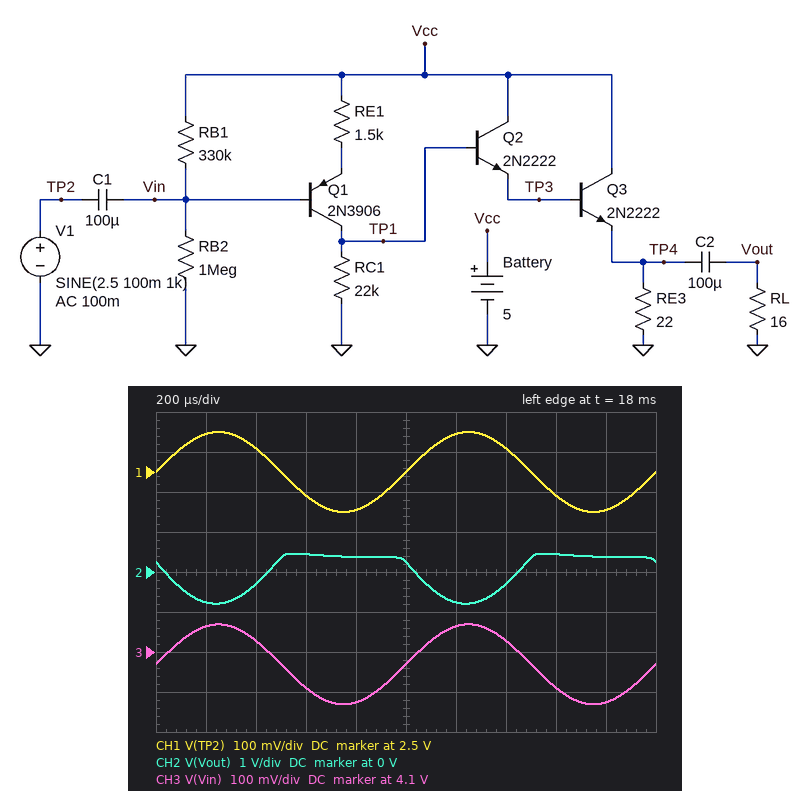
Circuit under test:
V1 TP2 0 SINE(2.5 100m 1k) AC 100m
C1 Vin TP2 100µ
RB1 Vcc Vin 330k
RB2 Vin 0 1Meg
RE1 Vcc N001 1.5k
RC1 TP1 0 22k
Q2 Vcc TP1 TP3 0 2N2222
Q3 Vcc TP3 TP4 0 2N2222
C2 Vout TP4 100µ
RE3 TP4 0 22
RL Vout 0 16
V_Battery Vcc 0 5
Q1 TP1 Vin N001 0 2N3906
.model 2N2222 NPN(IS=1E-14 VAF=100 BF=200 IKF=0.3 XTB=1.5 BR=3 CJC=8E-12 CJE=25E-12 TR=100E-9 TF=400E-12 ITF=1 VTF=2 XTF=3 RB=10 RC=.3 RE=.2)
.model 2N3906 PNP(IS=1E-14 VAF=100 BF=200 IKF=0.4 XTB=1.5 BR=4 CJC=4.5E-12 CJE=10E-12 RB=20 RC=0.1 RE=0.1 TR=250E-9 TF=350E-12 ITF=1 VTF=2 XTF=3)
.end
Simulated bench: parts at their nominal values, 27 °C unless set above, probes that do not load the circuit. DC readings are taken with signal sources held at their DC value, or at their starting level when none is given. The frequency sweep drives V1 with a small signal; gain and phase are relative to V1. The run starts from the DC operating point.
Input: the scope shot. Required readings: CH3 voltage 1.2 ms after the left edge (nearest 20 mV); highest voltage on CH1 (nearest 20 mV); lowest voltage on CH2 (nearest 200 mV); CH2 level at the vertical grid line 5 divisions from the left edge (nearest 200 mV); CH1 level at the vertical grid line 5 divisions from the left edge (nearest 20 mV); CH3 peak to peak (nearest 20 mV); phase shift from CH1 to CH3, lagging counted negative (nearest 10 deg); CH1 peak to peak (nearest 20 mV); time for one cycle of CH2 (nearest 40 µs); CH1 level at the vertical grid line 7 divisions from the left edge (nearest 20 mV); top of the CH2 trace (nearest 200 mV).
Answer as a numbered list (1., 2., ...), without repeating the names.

1. 4.16 V
2. 2.60 V
3. -800 mV
4. 200 mV
5. 2.50 V
6. 200 mV
7. 0 deg
8. 200 mV
9. 1.00 ms
10. 2.56 V
11. 400 mV
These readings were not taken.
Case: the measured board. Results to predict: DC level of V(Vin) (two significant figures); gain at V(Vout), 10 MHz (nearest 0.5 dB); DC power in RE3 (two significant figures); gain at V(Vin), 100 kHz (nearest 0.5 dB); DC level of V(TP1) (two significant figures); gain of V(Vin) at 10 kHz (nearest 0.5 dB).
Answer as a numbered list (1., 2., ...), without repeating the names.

1. 4.1 V
2. -3.5 dB
3. 420 mW
4. 0 dB
5. 4.5 V
6. 0 dB
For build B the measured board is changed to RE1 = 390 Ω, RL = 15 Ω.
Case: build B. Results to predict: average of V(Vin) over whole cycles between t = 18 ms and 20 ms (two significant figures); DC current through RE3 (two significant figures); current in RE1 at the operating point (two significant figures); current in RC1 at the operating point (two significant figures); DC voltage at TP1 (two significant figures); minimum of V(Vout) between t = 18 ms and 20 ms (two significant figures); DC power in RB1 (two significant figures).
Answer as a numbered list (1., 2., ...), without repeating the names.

1. 4.3 V
2. 150 mA
3. 230 µA
4. 220 µA
5. 4.8 V
6. -1.1 V
7. 1.5 µW
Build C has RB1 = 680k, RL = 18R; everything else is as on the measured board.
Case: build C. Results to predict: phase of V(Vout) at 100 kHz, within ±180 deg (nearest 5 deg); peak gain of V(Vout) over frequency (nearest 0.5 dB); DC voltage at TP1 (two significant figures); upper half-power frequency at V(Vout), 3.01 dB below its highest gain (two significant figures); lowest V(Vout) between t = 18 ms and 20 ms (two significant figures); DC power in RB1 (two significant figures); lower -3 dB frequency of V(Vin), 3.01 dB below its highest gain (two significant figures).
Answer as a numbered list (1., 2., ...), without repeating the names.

1. 155 deg
2. 11.5 dB
3. 4.6 V
4. 280 kHz
5. -770 mV
6. 1.3 µW
7. 520 mHz
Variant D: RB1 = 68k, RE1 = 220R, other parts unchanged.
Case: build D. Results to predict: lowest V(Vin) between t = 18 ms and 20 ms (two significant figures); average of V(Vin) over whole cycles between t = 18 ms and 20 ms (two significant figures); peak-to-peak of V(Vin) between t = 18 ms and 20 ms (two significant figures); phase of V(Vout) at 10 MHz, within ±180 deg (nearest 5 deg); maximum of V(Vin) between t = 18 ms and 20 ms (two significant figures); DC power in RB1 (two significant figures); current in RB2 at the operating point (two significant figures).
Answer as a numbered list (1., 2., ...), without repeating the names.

1. 4.6 V
2. 4.7 V
3. 200 mV
4. 90 deg
5. 4.8 V
6. 1.5 µW
7. 4.7 µA
